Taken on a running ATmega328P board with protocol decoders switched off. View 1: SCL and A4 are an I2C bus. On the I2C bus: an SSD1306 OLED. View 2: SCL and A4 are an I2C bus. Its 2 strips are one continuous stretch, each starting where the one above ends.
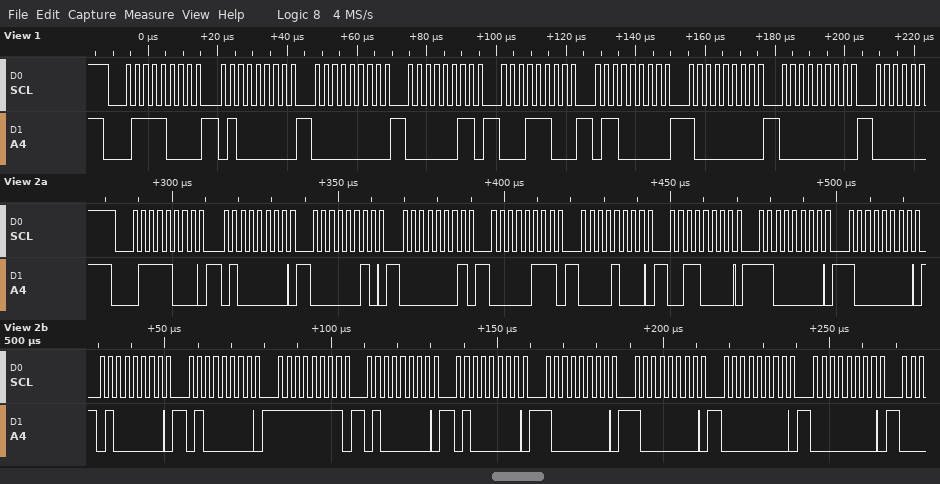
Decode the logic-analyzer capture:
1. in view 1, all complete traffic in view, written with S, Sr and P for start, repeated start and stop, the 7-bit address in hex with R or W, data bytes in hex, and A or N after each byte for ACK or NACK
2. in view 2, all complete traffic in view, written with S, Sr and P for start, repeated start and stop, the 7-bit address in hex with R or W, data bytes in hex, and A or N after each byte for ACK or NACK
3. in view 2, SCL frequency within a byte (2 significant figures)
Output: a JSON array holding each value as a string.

["S 3CW A 40 A 00 A 03 A 1C A 60 A 80 A 00 A", "S 3CW A 40 A 02 A 01 A 07 A 08 A 30 A C0 A 80 A 40 A 40 A FF A 40 A 40 A 80 A 80 A 00 A 00 A", "400 kHz"]
